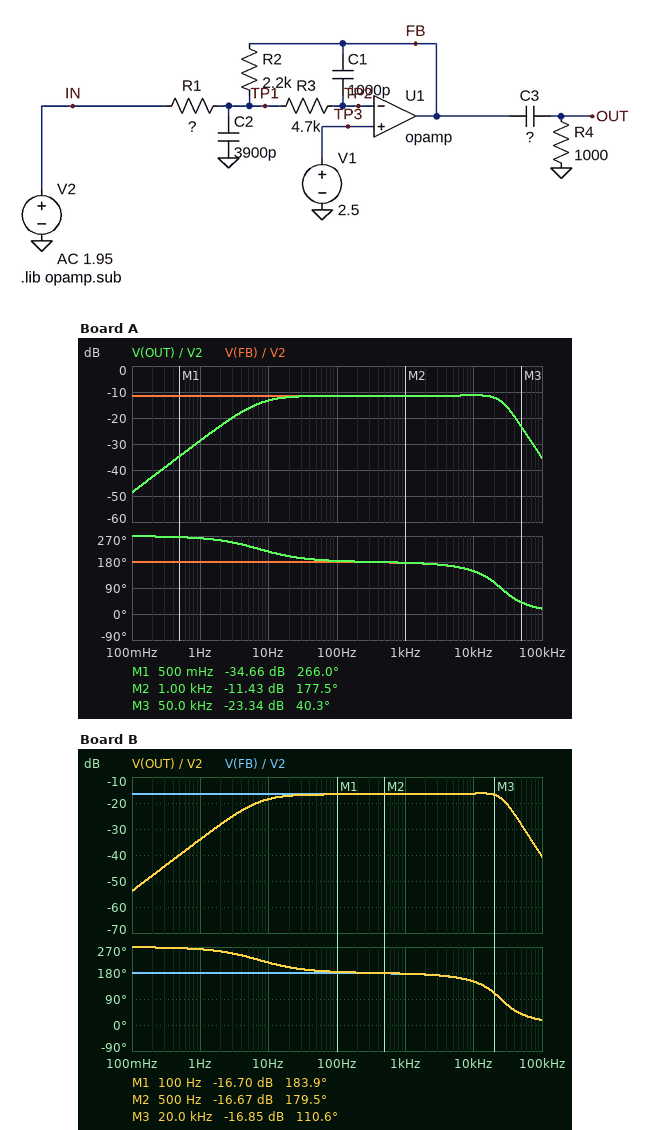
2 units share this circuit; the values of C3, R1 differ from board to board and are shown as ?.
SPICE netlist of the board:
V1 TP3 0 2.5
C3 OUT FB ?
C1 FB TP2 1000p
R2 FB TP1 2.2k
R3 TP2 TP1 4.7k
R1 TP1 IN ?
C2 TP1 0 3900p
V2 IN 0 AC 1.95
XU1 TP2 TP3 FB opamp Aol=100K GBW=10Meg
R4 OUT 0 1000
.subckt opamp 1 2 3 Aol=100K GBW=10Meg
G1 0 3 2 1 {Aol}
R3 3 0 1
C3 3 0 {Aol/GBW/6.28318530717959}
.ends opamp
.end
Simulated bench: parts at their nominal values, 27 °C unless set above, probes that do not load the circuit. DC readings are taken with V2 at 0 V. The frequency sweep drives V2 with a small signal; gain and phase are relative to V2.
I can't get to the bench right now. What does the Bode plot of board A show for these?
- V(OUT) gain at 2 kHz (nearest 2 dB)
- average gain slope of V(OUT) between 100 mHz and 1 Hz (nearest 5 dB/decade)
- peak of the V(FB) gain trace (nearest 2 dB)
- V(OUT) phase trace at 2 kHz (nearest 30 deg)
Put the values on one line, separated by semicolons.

-12 dB; 20 dB/decade; -12 dB; 180 deg
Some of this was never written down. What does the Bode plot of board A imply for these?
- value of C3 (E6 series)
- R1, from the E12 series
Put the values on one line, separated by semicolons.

22 µF; 8.2 kΩ
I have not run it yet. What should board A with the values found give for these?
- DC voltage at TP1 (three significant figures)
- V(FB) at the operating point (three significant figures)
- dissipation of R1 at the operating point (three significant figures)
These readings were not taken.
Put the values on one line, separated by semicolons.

2.50 V; 3.17 V; 762 µW
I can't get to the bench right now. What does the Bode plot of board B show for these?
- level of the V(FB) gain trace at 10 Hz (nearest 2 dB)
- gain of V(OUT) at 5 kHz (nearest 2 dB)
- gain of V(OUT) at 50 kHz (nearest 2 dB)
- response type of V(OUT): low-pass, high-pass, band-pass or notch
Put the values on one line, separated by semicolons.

-16 dB; -16 dB; -28 dB; band-pass
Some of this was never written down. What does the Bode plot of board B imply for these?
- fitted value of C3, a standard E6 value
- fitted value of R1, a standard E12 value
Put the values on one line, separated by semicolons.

22 µF; 15 kΩ
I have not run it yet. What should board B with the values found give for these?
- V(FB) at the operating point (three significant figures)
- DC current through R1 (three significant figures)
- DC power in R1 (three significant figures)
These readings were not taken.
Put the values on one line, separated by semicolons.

2.87 V; 167 µA; 417 µW
